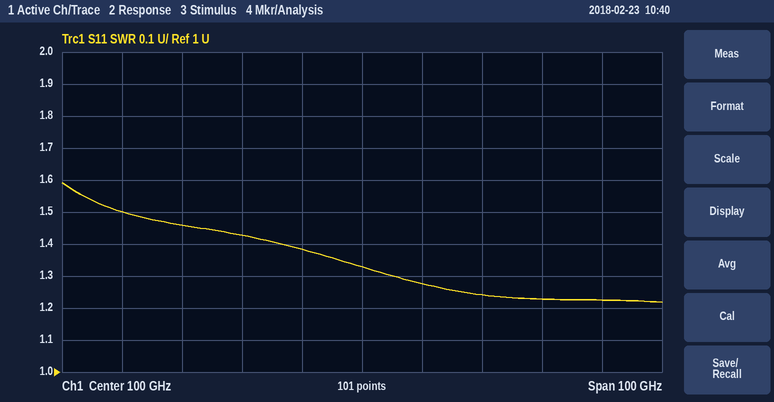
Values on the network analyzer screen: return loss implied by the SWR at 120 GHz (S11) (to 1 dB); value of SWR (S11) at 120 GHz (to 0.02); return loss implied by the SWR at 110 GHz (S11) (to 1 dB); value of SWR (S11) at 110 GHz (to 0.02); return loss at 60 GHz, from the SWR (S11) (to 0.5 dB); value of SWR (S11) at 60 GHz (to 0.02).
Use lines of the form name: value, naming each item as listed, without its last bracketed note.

return loss implied by the SWR at 120 GHz (S11): 19 dB
value of SWR (S11) at 120 GHz: 1.24
return loss implied by the SWR at 110 GHz (S11): 18 dB
value of SWR (S11) at 110 GHz: 1.28
return loss at 60 GHz, from the SWR (S11): 14.0 dB
value of SWR (S11) at 60 GHz: 1.50
